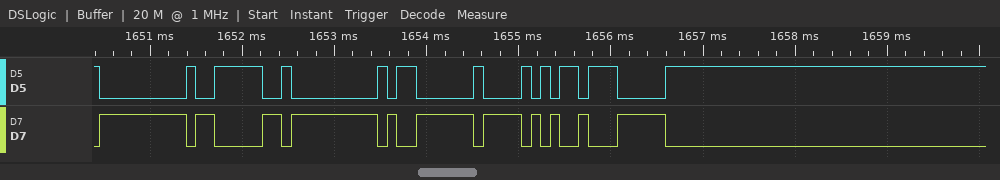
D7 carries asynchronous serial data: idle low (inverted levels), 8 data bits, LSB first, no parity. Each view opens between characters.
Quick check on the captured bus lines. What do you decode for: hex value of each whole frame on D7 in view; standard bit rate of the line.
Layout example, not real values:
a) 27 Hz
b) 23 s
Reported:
a) 00, 3E, 00, 03, A8, 07
b) 9600 baud
